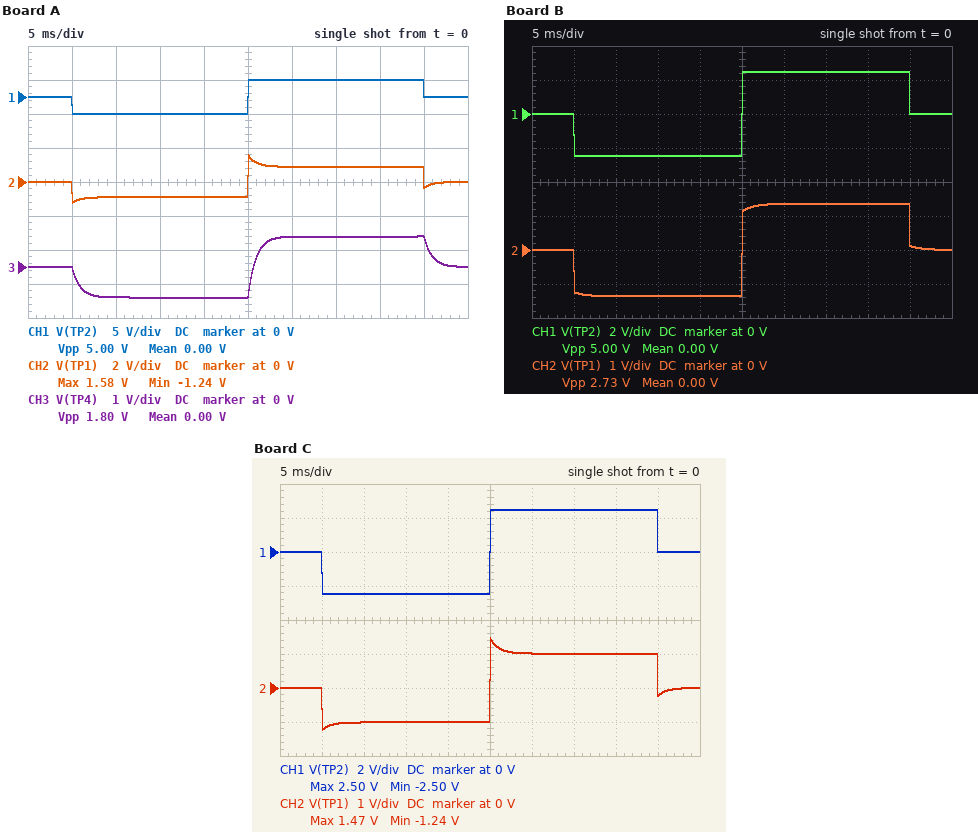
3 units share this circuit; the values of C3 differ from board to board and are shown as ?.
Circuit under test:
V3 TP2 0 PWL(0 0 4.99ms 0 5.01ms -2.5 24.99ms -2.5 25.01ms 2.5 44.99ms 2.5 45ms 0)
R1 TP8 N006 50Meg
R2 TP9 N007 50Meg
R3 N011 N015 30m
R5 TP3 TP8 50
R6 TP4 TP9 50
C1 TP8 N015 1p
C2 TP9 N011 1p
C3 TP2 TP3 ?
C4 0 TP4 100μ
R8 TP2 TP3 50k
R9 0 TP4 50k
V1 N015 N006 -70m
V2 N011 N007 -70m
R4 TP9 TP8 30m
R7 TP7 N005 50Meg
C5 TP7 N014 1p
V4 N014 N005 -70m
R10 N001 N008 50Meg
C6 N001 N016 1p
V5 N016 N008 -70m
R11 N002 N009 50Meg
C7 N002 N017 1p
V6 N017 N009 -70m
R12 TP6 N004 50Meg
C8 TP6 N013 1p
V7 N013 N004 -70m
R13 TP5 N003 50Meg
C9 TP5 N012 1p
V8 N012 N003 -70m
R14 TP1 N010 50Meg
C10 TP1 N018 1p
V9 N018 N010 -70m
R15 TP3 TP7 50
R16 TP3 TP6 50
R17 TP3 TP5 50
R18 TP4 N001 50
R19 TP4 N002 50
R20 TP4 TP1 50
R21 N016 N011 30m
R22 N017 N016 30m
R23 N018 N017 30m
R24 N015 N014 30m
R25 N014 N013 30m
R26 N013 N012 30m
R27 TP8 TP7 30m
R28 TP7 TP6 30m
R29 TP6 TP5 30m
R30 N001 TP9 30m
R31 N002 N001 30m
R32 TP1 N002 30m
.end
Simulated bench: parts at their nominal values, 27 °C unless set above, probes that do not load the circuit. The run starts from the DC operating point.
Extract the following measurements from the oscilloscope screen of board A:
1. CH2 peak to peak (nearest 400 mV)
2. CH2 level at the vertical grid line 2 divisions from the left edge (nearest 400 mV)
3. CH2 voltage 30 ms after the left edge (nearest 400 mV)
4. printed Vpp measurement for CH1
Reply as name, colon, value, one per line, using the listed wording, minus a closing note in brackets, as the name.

CH2 peak to peak: 2.8 V
CH2 level at the vertical grid line 2 divisions from the left edge: -800 mV
CH2 voltage 30 ms after the left edge: 800 mV
printed Vpp measurement for CH1: 5.00 V
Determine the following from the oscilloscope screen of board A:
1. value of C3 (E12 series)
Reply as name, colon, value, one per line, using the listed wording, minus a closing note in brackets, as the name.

value of C3: 56 µF
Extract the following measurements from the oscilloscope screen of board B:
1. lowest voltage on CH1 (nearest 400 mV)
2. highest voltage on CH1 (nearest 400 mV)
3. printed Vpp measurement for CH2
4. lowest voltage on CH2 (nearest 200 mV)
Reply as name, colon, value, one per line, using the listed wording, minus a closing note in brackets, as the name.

lowest voltage on CH1: -2.4 V
highest voltage on CH1: 2.4 V
printed Vpp measurement for CH2: 2.73 V
lowest voltage on CH2: -1.4 V
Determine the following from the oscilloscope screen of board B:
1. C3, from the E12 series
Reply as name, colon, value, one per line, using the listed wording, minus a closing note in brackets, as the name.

C3, from the E12 series: 120 µF
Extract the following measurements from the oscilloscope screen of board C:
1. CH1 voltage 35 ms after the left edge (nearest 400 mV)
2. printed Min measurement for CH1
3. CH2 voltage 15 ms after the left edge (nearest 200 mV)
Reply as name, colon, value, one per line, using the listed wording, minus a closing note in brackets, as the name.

CH1 voltage 35 ms after the left edge: 2.4 V
printed Min measurement for CH1: -2.50 V
CH2 voltage 15 ms after the left edge: -1.0 V
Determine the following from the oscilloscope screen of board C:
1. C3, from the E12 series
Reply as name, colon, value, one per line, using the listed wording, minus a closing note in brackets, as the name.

C3, from the E12 series: 68 µF
